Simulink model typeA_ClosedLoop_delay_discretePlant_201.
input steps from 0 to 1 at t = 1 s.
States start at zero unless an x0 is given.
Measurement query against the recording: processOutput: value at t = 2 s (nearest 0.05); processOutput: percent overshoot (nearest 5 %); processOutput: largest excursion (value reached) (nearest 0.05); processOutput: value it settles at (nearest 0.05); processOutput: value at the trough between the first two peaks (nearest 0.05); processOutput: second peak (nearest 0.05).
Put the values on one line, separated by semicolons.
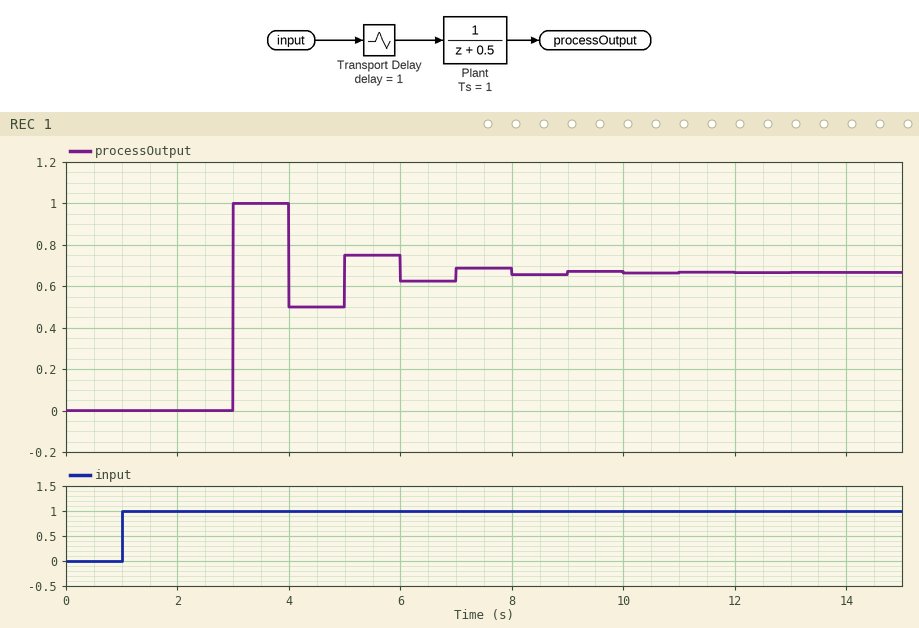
0.00; 50 %; 1.00; 0.65; 0.50; 0.75
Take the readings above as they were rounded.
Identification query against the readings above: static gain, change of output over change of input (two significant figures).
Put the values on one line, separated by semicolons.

0.65
